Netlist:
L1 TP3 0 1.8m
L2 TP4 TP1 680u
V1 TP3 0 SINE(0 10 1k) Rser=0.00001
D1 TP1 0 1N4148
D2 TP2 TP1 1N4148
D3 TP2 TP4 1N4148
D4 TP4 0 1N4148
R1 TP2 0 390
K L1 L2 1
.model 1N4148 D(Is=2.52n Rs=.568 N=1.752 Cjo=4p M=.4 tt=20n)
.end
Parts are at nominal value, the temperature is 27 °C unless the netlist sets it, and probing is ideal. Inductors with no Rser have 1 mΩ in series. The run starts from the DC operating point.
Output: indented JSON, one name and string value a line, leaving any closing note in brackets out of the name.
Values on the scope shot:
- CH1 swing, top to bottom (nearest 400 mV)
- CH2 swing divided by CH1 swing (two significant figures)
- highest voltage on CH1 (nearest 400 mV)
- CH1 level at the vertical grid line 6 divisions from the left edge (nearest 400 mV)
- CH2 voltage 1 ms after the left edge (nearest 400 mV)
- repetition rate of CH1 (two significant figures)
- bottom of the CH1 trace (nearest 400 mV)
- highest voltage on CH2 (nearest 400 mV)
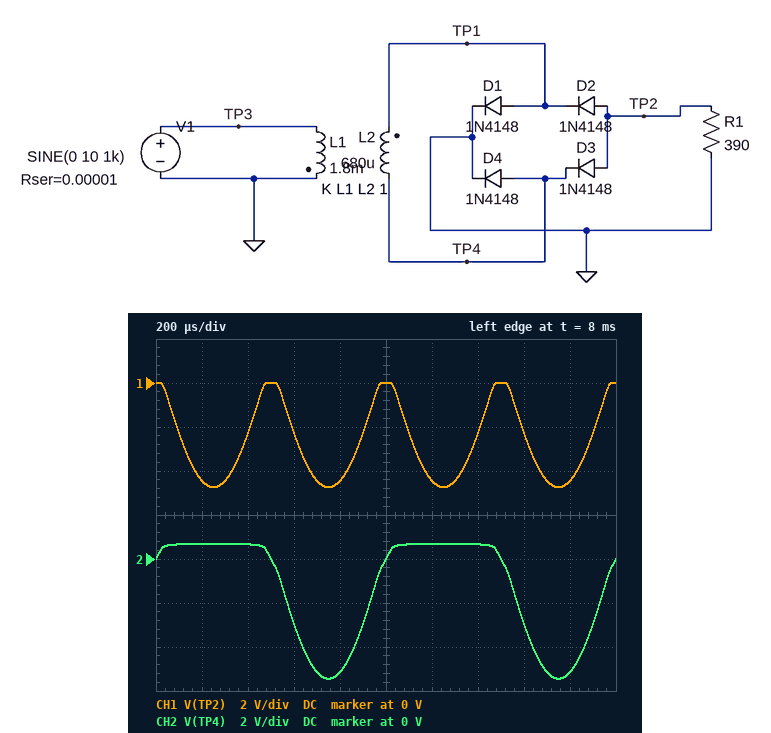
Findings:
{
  "CH1 swing, top to bottom": "4.8 V",
  "CH2 swing divided by CH1 swing": "1.3",
  "highest voltage on CH1": "0 V",
  "CH1 level at the vertical grid line 6 divisions from the left edge": "-4.4 V",
  "CH2 voltage 1 ms after the left edge": "0 V",
  "repetition rate of CH1": "2.0 kHz",
  "bottom of the CH1 trace": "-4.8 V",
  "highest voltage on CH2": "800 mV"
}
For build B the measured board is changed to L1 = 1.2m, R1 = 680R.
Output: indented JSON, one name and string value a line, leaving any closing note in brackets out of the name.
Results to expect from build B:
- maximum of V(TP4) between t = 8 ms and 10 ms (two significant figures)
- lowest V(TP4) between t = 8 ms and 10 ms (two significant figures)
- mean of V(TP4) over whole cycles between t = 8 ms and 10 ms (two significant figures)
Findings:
{
  "maximum of V(TP4) between t = 8 ms and 10 ms": "690 mV",
  "lowest V(TP4) between t = 8 ms and 10 ms": "-6.8 V",
  "mean of V(TP4) over whole cycles between t = 8 ms and 10 ms": "-1.8 V"
}
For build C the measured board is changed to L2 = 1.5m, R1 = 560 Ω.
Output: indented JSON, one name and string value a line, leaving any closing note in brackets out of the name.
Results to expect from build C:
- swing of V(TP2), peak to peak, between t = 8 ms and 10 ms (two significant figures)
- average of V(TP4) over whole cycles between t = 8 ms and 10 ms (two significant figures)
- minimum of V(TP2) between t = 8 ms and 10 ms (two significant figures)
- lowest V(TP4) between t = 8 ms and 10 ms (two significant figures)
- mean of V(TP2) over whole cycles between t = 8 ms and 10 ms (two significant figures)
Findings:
{
  "swing of V(TP2), peak to peak, between t = 8 ms and 10 ms": "7.7 V",
  "average of V(TP4) over whole cycles between t = 8 ms and 10 ms": "-2.3 V",
  "minimum of V(TP2) between t = 8 ms and 10 ms": "-7.7 V",
  "lowest V(TP4) between t = 8 ms and 10 ms": "-8.4 V",
  "mean of V(TP2) over whole cycles between t = 8 ms and 10 ms": "-4.5 V"
}
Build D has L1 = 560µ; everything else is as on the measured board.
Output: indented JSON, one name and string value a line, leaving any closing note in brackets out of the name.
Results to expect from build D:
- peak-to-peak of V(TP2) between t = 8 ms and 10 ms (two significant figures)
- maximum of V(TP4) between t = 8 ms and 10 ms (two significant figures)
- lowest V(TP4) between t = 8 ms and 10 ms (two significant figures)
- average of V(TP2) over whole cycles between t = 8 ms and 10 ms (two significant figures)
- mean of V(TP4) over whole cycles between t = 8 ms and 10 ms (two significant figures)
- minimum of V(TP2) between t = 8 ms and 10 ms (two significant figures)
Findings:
{
  "peak-to-peak of V(TP2) between t = 8 ms and 10 ms": "9.5 V",
  "maximum of V(TP4) between t = 8 ms and 10 ms": "740 mV",
  "lowest V(TP4) between t = 8 ms and 10 ms": "-10 V",
  "average of V(TP2) over whole cycles between t = 8 ms and 10 ms": "-5.7 V",
  "mean of V(TP4) over whole cycles between t = 8 ms and 10 ms": "-2.8 V",
  "minimum of V(TP2) between t = 8 ms and 10 ms": "-9.5 V"
}
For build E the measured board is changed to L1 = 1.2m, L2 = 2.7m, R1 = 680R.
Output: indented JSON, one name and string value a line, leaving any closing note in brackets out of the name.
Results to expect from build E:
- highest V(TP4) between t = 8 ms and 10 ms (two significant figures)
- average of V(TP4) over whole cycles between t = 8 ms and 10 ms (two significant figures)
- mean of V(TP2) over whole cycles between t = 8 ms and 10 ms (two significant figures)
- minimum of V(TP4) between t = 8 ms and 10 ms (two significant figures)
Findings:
{
  "highest V(TP4) between t = 8 ms and 10 ms": "730 mV",
  "average of V(TP4) over whole cycles between t = 8 ms and 10 ms": "-4.1 V",
  "mean of V(TP2) over whole cycles between t = 8 ms and 10 ms": "-8.2 V",
  "minimum of V(TP4) between t = 8 ms and 10 ms": "-14 V"
}
